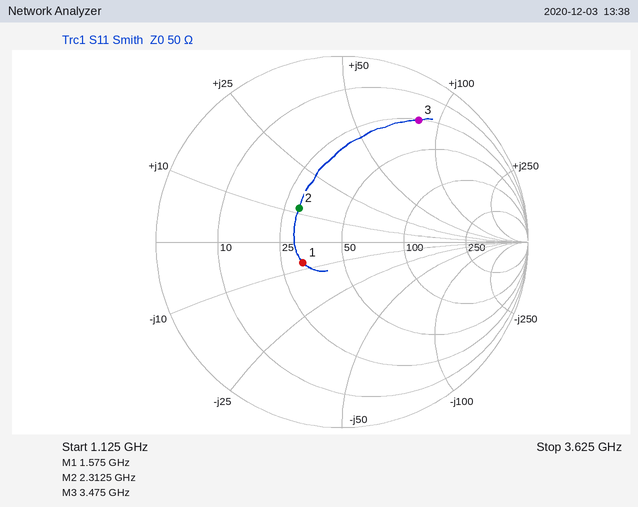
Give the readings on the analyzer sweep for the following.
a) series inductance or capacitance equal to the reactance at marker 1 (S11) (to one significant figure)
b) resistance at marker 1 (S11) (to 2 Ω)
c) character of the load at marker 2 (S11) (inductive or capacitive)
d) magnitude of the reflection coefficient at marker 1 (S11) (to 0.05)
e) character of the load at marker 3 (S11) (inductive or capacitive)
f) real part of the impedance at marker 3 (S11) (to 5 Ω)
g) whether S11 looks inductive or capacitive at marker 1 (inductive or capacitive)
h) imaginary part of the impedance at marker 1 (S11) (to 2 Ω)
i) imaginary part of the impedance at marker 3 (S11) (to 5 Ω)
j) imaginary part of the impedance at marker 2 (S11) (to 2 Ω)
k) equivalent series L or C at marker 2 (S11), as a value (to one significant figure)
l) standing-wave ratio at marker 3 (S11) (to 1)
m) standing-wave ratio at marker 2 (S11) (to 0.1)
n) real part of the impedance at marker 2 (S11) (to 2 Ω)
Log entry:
10 pF
32 Ω
inductive
0.25
inductive
25 Ω
capacitive
-8 Ω
+85 Ω
+12 Ω
800 pH
8
1.8
30 Ω
